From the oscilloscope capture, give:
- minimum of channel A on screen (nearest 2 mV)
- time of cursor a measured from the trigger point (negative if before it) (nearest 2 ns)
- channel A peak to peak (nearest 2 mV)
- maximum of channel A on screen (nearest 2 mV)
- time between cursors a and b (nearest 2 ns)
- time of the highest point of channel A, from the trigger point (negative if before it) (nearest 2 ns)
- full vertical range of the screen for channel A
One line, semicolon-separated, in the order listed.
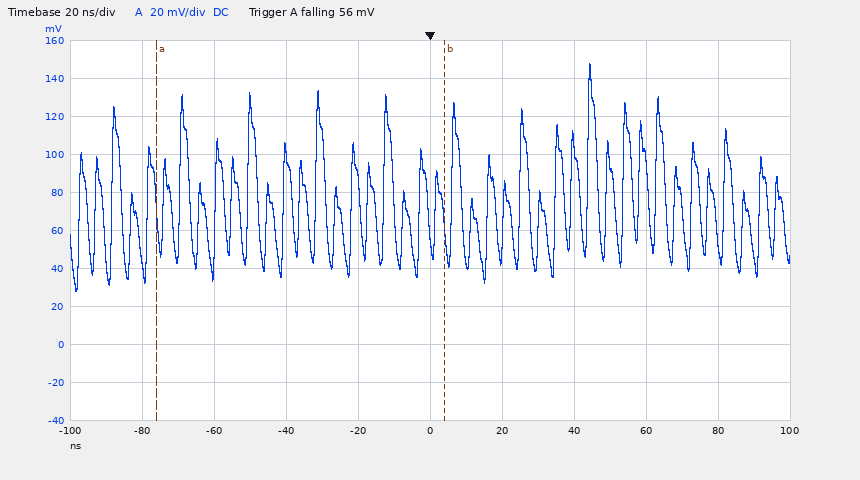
28 mV; -76 ns; 120 mV; 148 mV; 80 ns; +44 ns; 200 mV
